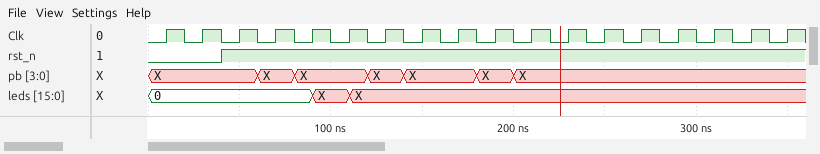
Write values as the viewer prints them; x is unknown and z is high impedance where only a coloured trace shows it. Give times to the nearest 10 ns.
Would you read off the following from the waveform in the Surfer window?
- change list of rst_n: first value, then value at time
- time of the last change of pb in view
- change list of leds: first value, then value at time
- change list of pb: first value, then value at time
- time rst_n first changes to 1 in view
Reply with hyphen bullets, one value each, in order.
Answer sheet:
- 0, 1 at 40 ns
- 200 ns
- 0, X at 90 ns, X at 110 ns
- X, X at 60 ns, X at 80 ns, X at 120 ns, X at 140 ns, X at 180 ns, X at 200 ns
- 40 ns
